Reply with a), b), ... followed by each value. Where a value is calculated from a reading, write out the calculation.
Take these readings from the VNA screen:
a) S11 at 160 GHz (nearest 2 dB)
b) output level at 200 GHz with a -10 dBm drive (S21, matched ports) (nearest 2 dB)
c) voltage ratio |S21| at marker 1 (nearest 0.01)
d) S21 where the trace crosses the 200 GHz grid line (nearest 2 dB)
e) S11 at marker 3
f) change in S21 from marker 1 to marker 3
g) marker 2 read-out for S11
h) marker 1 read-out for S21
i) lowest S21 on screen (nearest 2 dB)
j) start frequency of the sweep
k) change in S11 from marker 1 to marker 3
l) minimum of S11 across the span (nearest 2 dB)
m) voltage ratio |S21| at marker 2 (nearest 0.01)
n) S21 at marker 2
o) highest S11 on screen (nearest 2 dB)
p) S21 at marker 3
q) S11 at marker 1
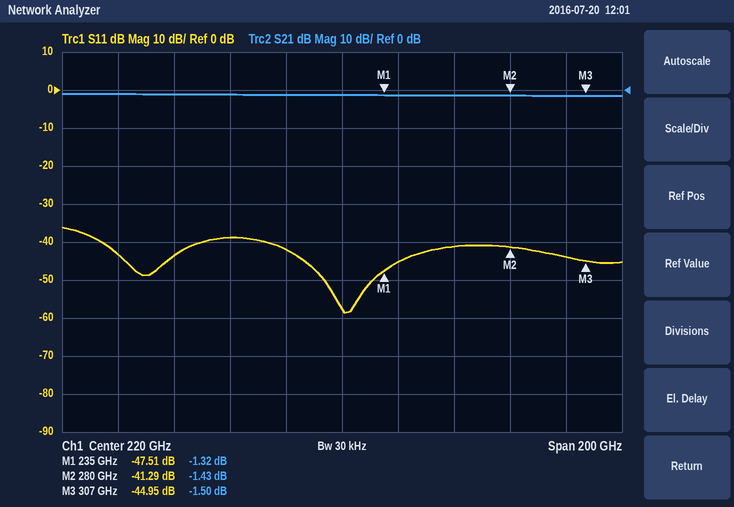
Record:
a) -44 dB
b) -10 dBm + (-2 dB) = -12 dBm
c) 10^(-1.32/20) ≈ 0.86
d) -2 dB
e) -44.95 dB
f) -1.5 − (-1.32) = -0.18 dB
g) -41.29 dB
h) -1.32 dB
i) -2 dB
j) 120 GHz
k) -44.95 − (-47.51) = 2.56 dB
l) -58 dB
m) 10^(-1.43/20) ≈ 0.85
n) -1.43 dB
o) -36 dB
p) -1.50 dB
q) -47.51 dB
